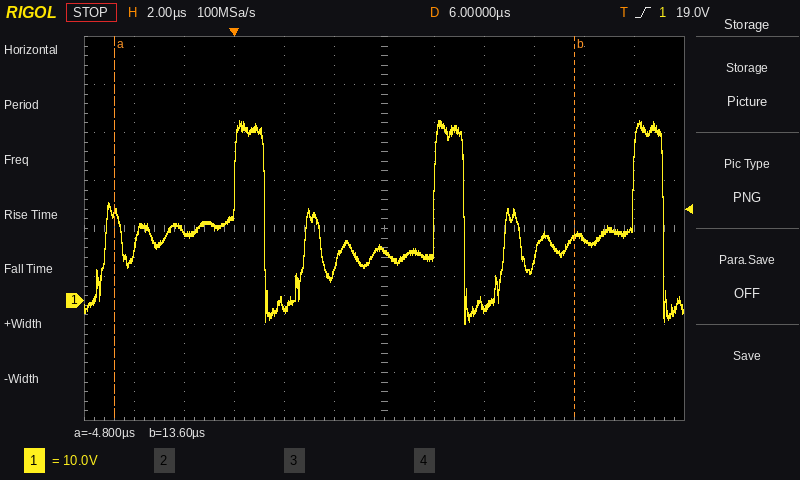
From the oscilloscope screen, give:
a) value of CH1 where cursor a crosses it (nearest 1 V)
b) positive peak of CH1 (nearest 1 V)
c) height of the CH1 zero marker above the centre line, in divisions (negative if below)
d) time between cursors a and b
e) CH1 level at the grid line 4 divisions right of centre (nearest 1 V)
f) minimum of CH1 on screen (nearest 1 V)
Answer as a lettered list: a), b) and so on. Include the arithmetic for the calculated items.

a) 18 V
b) 38 V
c) -1.5 div
d) 13.6 µs − (-4.8 µs) = 18.4 µs
e) 13 V
f) -5 V
